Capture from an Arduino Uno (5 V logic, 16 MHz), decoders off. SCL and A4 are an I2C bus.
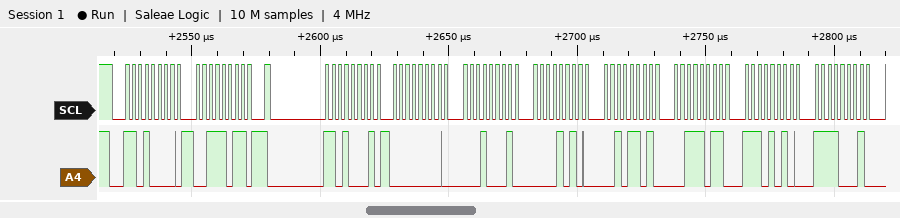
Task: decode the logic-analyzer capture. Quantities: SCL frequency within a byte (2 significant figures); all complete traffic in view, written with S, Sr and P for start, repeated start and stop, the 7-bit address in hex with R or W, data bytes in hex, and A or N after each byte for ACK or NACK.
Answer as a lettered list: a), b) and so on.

a) 400 kHz
b) S 68W A 3B A Sr 68R A 00 A 11 A 0A A 2D A 3B A EA A F1 A
